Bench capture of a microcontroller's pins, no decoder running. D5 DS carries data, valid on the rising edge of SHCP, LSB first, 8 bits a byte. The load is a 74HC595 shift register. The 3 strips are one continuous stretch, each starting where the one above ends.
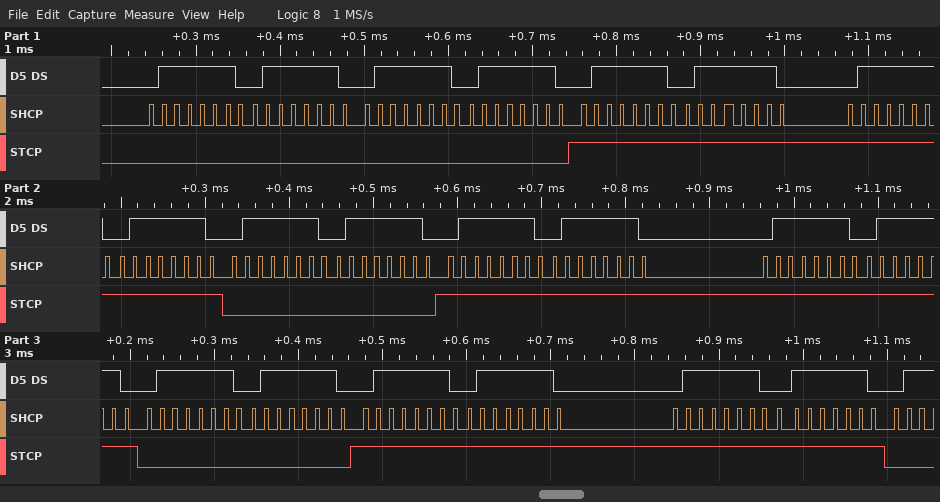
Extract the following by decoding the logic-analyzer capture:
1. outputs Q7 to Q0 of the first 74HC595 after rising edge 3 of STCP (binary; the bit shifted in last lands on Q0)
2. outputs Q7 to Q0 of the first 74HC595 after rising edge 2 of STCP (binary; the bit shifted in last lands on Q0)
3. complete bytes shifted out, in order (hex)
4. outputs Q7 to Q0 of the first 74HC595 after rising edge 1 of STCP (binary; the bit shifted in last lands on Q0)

01111110
01111110
7E 7E 7E 7E 7E 7E 7E 7E 7E 7E 7E 7E 7E 7E 7E 7E 7E 7E 7E 7E
01111110
